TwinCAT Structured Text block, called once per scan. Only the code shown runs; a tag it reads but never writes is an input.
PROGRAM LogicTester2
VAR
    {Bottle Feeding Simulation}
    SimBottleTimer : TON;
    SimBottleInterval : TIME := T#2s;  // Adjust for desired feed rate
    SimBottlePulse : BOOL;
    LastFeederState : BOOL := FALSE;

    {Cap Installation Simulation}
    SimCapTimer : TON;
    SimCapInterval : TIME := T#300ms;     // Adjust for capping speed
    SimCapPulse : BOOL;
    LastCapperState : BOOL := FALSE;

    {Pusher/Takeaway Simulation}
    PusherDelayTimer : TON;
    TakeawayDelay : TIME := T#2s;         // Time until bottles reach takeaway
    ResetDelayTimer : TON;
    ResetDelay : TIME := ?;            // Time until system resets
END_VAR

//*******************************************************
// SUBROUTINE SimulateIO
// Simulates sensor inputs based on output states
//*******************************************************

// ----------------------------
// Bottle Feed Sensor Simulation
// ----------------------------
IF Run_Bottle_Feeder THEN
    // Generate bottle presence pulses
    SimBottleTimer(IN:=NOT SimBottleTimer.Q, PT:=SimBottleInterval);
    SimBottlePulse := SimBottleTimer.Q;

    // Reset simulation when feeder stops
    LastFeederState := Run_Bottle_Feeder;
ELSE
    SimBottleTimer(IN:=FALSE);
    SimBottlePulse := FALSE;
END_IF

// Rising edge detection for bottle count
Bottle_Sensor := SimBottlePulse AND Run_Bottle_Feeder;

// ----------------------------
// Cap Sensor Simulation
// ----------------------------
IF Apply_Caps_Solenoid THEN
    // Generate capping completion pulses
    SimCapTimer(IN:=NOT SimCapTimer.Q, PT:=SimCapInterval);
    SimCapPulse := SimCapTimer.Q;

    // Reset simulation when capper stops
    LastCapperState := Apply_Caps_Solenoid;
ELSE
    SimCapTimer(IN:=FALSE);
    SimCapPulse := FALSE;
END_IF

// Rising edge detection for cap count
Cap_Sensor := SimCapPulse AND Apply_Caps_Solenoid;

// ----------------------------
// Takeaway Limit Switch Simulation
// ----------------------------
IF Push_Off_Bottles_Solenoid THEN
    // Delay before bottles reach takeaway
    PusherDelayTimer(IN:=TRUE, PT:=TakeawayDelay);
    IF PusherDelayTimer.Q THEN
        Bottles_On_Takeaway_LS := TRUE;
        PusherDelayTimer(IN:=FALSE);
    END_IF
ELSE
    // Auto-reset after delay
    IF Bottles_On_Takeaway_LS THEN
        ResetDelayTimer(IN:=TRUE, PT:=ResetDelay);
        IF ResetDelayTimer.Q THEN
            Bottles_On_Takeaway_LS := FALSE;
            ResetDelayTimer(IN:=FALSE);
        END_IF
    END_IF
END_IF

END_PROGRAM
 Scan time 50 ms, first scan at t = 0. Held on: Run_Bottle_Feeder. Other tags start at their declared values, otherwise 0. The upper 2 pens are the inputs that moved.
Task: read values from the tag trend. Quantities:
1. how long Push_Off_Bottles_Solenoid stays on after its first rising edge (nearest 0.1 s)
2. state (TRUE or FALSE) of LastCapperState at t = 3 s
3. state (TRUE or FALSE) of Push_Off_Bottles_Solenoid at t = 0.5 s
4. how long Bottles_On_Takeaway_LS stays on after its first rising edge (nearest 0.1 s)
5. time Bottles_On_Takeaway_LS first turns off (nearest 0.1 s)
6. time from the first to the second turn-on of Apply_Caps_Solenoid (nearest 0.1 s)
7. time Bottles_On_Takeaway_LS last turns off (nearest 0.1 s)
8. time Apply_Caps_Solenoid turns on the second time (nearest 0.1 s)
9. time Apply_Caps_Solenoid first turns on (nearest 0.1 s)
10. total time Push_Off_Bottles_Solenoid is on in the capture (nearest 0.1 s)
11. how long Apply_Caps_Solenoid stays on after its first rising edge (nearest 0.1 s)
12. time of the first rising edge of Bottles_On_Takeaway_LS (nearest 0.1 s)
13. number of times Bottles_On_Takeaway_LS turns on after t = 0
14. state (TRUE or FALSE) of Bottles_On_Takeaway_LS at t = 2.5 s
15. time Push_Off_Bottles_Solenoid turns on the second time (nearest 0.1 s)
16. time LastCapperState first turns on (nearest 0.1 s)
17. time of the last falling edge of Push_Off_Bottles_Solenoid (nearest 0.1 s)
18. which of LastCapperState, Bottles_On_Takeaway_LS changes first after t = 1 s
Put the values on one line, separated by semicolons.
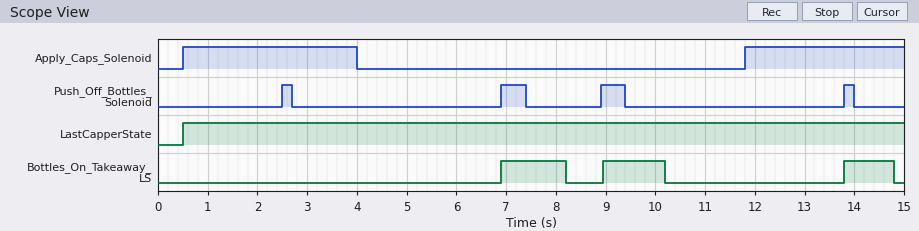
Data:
0.2 s; TRUE; FALSE; 1.3 s; 8.2 s; 11.3 s; 14.8 s; 11.8 s; 0.5 s; 1.4 s; 3.5 s; 6.9 s; 3; FALSE; 6.9 s; 0.5 s; 14.0 s; Bottles_On_Takeaway_LS
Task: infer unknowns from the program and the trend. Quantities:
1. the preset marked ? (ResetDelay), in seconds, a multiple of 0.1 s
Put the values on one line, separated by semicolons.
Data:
0.8 s
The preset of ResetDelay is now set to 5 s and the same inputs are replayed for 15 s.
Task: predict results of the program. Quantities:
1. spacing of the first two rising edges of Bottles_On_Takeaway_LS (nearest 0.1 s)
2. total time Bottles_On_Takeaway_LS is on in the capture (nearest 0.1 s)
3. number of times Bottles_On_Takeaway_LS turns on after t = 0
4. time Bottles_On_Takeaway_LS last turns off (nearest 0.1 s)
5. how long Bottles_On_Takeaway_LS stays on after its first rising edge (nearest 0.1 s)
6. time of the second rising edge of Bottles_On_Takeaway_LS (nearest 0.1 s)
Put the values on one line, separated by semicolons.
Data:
6.9 s; 6.7 s; 2; 12.4 s; 5.5 s; 13.8 s
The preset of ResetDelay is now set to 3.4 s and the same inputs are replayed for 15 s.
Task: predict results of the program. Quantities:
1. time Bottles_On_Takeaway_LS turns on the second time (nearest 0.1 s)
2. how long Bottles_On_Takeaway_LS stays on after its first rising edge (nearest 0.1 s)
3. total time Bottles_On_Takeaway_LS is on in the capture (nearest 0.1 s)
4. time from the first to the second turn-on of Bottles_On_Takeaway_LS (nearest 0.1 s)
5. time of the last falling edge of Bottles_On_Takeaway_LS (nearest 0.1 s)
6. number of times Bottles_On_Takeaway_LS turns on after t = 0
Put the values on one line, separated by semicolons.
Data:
13.8 s; 3.9 s; 5.1 s; 6.9 s; 10.8 s; 2
